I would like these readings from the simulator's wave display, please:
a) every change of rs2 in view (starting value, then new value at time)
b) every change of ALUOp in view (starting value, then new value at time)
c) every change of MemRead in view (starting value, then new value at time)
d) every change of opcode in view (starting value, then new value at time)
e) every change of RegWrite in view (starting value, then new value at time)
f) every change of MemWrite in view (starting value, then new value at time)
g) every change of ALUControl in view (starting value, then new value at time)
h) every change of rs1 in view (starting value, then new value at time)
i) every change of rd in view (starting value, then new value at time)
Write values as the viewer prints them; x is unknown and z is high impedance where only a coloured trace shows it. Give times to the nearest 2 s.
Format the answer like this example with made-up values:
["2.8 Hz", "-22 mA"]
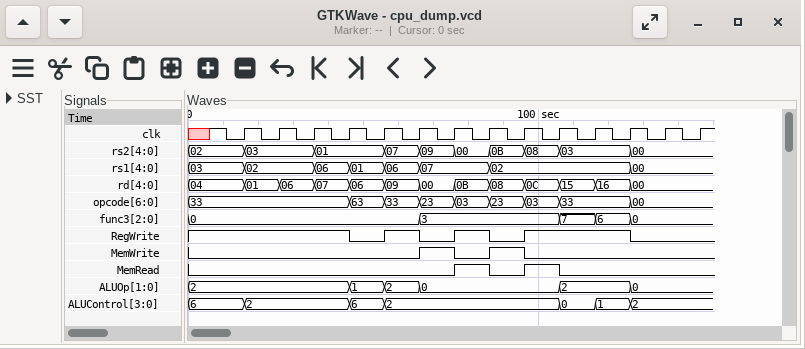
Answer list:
["02, 03 at 16 s, 01 at 36 s, 07 at 56 s, 09 at 66 s, 00 at 76 s, 0B at 86 s, 08 at 96 s, 03 at 106 s, 00 at 126 s", "2, 1 at 46 s, 2 at 56 s, 0 at 66 s, 2 at 106 s, 0 at 126 s", "0, 1 at 76 s, 0 at 86 s, 1 at 96 s, 0 at 106 s", "33, 63 at 46 s, 33 at 56 s, 23 at 66 s, 03 at 76 s, 23 at 86 s, 03 at 96 s, 33 at 106 s, 00 at 126 s", "1, 0 at 46 s, 1 at 56 s, 0 at 66 s, 1 at 76 s, 0 at 86 s, 1 at 96 s, 0 at 126 s", "0, 1 at 66 s, 0 at 76 s, 1 at 86 s, 0 at 96 s", "6, 2 at 16 s, 6 at 46 s, 2 at 56 s, 0 at 106 s, 1 at 116 s, 2 at 126 s", "03, 02 at 16 s, 06 at 36 s, 01 at 46 s, 06 at 56 s, 07 at 66 s, 02 at 86 s, 00 at 126 s", "04, 01 at 16 s, 06 at 26 s, 07 at 36 s, 06 at 46 s, 09 at 56 s, 00 at 66 s, 0B at 76 s, 08 at 86 s, 0C at 96 s, 15 at 106 s, 16 at 116 s, 00 at 126 s"]
